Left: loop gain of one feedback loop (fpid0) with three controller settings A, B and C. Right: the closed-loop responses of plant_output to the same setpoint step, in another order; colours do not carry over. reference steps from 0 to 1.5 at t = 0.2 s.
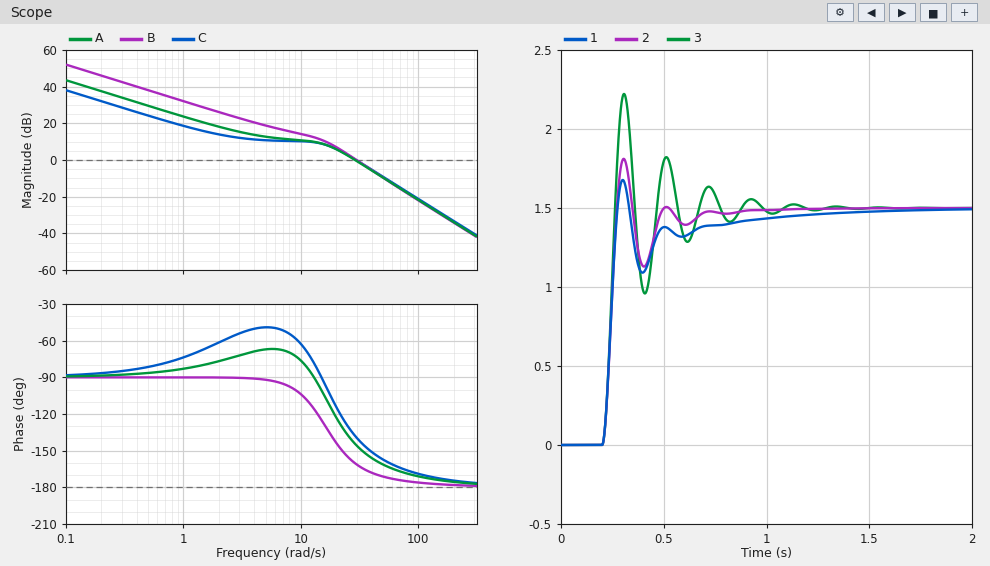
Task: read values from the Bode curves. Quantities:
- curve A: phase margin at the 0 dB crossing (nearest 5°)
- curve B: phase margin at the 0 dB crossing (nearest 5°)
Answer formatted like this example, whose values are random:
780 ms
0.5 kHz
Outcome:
35°
20°
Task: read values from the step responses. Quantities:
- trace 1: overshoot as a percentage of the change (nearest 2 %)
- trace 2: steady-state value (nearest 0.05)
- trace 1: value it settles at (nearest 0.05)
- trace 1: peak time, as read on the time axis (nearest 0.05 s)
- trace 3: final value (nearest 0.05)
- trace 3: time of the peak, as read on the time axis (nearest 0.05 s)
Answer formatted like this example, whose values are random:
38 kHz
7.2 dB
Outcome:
12 %
1.50
1.50
0.30 s
1.50
0.30 s
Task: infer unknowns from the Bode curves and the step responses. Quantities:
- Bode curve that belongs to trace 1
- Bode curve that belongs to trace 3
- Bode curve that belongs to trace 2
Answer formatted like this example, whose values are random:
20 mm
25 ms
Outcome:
C
B
A
